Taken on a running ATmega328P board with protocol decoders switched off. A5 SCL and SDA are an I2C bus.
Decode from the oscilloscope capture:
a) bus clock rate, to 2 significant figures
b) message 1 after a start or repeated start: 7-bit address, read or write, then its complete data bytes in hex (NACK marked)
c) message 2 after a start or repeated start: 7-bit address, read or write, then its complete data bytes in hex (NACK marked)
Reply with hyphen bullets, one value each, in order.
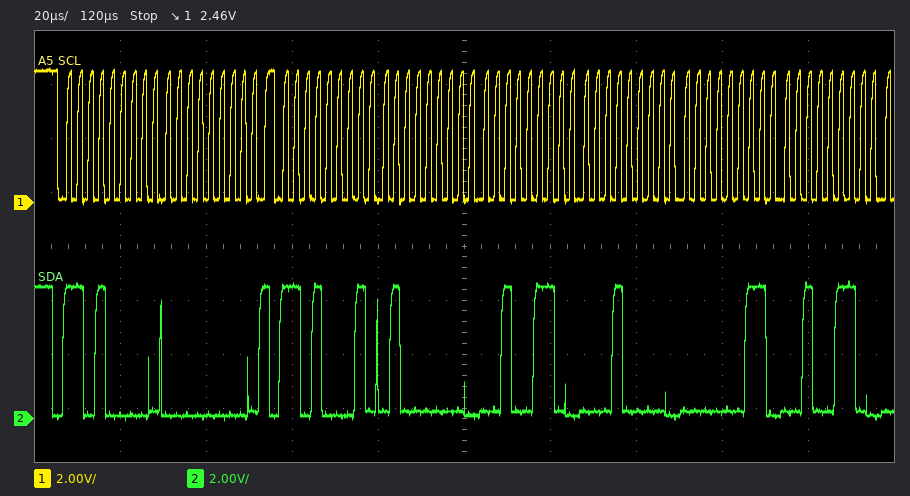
- 400 kHz
- 0x68 write: 00
- 0x68 read: 40 26 10 03 26
